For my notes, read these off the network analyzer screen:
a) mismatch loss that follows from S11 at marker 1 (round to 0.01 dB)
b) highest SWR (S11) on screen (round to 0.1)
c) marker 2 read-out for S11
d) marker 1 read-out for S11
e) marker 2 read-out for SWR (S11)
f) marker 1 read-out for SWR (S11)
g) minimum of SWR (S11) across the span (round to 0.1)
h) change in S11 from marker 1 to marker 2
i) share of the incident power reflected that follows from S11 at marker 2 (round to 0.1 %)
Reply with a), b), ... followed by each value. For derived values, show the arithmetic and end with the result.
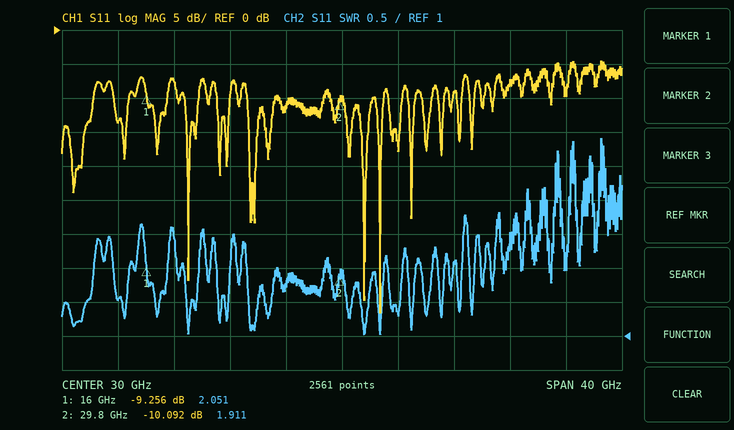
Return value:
a) −10 log10(1 − 10^(-9.256/10)) ≈ 0.55 dB
b) 3.9
c) -10.092 dB
d) -9.256 dB
e) 1.911
f) 2.051
g) 1.0
h) -10.092 − (-9.256) = -0.836 dB
i) 10^(-10.092/10) ≈ 9.8 %
